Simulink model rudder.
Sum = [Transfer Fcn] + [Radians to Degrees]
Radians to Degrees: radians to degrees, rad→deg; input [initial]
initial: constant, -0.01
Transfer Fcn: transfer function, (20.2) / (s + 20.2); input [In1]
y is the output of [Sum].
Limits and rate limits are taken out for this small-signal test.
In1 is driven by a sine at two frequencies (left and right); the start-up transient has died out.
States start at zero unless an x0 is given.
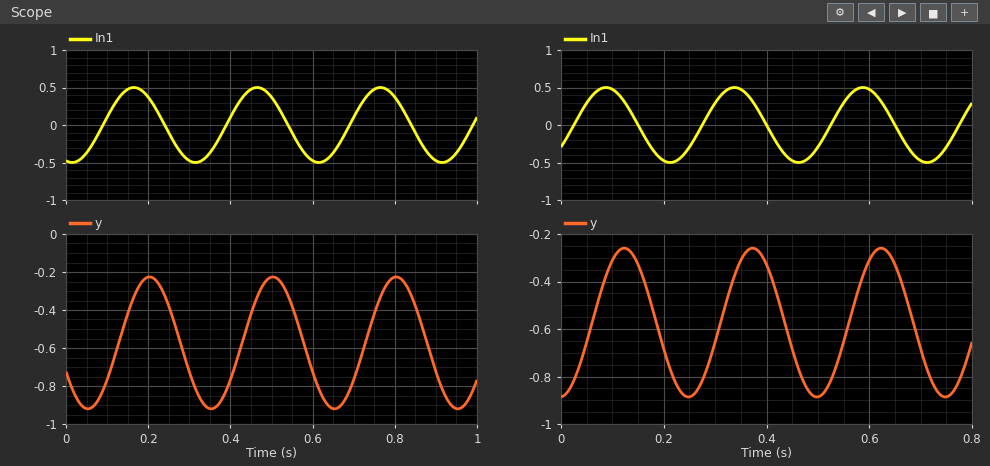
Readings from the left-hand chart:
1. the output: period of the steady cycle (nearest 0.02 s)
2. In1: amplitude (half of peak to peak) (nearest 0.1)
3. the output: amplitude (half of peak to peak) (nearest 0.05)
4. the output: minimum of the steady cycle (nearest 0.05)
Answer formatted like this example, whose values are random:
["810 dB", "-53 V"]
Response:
["0.30 s", "0.5", "0.35", "-0.90"]
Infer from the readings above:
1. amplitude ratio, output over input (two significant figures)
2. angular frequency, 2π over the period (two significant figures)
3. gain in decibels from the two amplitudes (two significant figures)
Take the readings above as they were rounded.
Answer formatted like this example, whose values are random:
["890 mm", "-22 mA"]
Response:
["0.70", "21 rad/s", "-3.1 dB"]
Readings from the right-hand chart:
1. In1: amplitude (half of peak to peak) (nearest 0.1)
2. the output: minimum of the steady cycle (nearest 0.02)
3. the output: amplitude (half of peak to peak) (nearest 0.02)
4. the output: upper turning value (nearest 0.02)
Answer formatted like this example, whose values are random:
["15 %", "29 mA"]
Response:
["0.5", "-0.88", "0.32", "-0.26"]
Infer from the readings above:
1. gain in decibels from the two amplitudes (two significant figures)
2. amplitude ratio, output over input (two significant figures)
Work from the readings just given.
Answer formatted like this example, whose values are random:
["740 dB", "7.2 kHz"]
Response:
["-3.9 dB", "0.64"]
